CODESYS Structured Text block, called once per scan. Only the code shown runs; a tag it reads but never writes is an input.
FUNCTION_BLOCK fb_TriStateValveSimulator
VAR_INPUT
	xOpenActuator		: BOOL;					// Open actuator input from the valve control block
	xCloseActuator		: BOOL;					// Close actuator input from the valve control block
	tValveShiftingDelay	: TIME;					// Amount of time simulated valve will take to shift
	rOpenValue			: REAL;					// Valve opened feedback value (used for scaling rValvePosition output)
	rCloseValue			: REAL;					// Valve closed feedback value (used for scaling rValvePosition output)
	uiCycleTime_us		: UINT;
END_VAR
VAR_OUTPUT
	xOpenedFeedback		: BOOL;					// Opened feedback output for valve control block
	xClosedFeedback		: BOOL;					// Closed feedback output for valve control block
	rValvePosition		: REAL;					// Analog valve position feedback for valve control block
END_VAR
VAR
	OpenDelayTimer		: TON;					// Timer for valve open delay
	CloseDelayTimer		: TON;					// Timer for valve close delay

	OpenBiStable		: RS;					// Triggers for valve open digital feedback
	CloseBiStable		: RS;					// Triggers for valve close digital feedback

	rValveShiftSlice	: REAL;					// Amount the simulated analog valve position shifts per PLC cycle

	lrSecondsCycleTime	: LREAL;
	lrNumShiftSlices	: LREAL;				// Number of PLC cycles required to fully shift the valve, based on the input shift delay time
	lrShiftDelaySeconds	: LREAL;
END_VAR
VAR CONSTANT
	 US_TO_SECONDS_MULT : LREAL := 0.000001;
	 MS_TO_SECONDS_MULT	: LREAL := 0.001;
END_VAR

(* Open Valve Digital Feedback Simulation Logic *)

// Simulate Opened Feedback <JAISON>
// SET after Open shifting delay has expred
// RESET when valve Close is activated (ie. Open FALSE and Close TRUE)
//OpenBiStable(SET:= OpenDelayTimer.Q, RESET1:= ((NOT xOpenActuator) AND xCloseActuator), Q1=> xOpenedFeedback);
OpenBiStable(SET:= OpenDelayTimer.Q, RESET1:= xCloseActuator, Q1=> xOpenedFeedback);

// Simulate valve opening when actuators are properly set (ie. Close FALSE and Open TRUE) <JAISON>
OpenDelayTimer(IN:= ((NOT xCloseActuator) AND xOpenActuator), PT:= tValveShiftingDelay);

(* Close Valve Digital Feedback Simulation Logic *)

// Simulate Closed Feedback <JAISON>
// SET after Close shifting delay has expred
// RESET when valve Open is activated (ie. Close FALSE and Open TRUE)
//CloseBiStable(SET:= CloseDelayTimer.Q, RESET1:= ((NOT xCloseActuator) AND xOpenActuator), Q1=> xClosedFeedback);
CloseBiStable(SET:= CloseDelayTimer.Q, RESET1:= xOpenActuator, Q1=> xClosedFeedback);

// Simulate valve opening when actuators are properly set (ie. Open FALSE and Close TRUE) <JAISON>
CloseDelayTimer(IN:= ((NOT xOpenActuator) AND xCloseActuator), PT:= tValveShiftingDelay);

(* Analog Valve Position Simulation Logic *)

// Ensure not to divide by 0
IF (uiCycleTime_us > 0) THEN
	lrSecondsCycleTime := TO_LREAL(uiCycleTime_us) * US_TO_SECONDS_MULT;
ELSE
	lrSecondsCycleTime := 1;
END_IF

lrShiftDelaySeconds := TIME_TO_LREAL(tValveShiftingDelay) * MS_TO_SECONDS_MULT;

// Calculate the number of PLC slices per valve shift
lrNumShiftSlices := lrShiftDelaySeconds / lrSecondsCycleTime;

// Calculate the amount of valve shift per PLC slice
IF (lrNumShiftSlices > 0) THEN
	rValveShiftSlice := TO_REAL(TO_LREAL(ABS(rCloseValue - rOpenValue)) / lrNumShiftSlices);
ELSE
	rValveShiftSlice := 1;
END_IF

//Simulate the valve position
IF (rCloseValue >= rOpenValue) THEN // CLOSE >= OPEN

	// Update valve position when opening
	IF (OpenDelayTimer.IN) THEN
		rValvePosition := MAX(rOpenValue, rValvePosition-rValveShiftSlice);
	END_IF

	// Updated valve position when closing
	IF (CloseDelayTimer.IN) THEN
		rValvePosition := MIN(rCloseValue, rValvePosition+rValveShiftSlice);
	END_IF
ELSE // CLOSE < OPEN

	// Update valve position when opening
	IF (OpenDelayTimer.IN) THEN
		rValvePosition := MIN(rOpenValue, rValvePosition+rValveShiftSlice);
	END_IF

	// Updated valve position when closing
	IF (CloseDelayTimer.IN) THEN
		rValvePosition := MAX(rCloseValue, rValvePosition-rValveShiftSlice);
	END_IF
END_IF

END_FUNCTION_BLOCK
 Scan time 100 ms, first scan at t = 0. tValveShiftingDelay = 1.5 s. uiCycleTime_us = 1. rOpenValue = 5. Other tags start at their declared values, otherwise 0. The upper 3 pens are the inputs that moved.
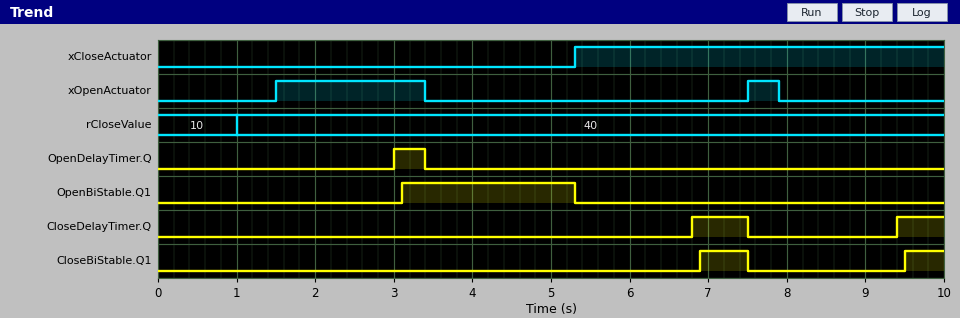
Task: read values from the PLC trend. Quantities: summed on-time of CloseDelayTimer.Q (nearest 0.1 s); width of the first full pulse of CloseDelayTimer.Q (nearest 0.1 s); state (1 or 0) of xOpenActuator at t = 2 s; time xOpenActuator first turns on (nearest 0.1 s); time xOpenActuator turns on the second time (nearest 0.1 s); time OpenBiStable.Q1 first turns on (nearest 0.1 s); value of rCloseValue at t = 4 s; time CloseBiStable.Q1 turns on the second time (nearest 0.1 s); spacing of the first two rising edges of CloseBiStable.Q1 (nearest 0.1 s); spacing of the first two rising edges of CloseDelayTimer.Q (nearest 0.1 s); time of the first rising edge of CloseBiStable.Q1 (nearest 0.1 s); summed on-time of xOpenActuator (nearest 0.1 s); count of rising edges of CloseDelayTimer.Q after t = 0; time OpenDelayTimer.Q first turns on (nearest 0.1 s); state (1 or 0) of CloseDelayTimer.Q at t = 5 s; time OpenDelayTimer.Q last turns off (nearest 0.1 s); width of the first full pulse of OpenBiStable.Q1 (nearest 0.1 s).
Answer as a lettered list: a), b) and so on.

a) 1.3 s
b) 0.7 s
c) 1
d) 1.5 s
e) 7.5 s
f) 3.1 s
g) 40
h) 9.5 s
i) 2.6 s
j) 2.6 s
k) 6.9 s
l) 2.3 s
m) 2
n) 3.0 s
o) 0
p) 3.4 s
q) 2.2 s
